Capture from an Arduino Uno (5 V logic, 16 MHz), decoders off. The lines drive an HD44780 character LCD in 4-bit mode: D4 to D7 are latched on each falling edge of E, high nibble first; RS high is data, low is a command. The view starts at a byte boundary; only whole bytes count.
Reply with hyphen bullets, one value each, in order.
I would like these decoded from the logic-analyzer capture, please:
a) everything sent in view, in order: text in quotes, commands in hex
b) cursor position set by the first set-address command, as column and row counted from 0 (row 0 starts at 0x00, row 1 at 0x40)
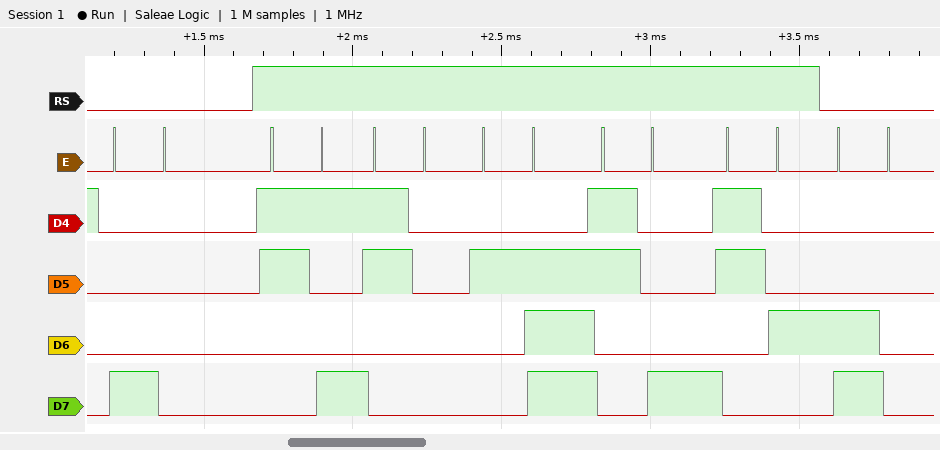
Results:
- 0x80 "90.84" 0xC0
- column 0, row 0
